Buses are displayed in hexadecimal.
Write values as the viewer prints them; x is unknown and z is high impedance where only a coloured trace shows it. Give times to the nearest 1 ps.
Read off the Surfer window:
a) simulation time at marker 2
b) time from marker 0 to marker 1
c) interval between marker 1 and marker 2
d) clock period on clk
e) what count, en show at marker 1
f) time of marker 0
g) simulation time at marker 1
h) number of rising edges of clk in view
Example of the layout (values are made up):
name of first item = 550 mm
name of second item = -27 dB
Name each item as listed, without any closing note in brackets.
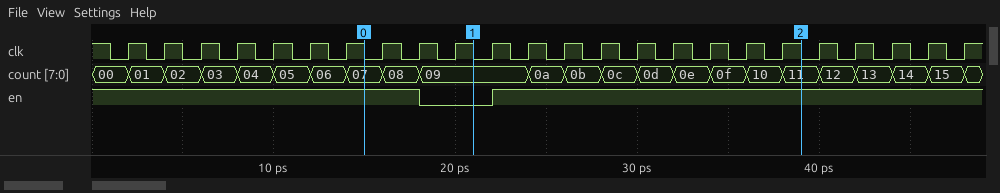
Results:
simulation time at marker 2 = 39 ps
time from marker 0 to marker 1 = 6 ps
interval between marker 1 and marker 2 = 18 ps
clock period on clk = 2 ps
what count, en show at marker 1 = count=09, en=0
time of marker 0 = 15 ps
simulation time at marker 1 = 21 ps
number of rising edges of clk in view = 24
